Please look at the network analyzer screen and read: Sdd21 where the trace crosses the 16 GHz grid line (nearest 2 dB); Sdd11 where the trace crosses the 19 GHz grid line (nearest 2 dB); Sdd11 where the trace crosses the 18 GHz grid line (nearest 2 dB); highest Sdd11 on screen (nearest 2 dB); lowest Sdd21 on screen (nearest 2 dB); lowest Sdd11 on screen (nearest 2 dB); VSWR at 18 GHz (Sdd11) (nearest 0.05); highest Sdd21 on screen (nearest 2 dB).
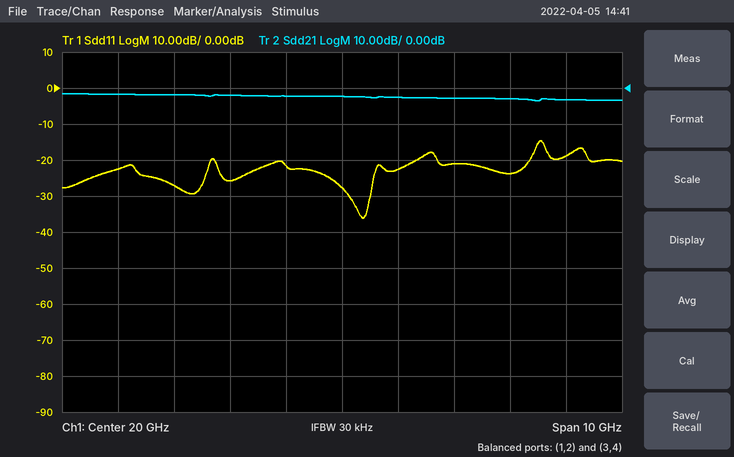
-2 dB
-22 dB
-26 dB
-14 dB
-4 dB
-36 dB
1.10
-2 dB
